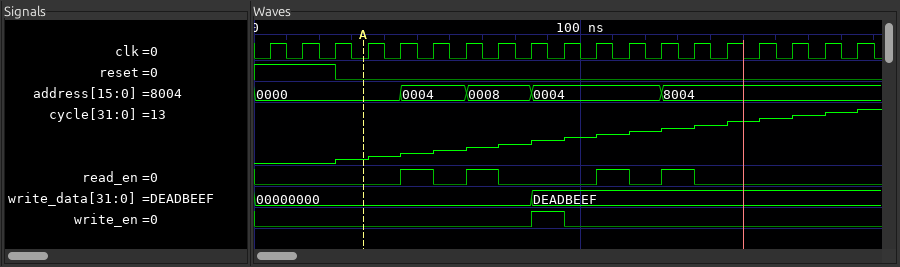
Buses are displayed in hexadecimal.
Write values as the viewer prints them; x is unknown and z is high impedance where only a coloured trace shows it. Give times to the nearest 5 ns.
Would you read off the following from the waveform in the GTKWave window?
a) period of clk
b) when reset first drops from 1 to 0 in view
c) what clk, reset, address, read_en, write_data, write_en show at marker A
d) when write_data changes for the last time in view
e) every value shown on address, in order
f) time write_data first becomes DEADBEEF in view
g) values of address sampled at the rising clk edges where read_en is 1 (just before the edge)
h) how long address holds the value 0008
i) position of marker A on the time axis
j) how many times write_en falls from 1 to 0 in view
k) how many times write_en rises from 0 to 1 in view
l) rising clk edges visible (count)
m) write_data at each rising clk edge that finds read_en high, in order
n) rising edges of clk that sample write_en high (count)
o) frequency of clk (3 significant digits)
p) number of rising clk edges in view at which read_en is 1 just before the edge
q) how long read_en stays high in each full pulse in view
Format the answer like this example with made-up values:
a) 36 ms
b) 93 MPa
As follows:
a) 10 ns
b) 25 ns
c) clk=0, reset=0, address=0000, read_en=0, write_data=00000000, write_en=0
d) 85 ns
e) 0000, 0004, 0008, 0004, 8004
f) 85 ns
g) 0004, 0008, 0004, 8004
h) 20 ns
i) 35 ns
j) 1
k) 1
l) 19
m) 00000000, 00000000, DEADBEEF, DEADBEEF
n) 1
o) 100 MHz
p) 4
q) 10 ns, 10 ns, 10 ns, 10 ns
